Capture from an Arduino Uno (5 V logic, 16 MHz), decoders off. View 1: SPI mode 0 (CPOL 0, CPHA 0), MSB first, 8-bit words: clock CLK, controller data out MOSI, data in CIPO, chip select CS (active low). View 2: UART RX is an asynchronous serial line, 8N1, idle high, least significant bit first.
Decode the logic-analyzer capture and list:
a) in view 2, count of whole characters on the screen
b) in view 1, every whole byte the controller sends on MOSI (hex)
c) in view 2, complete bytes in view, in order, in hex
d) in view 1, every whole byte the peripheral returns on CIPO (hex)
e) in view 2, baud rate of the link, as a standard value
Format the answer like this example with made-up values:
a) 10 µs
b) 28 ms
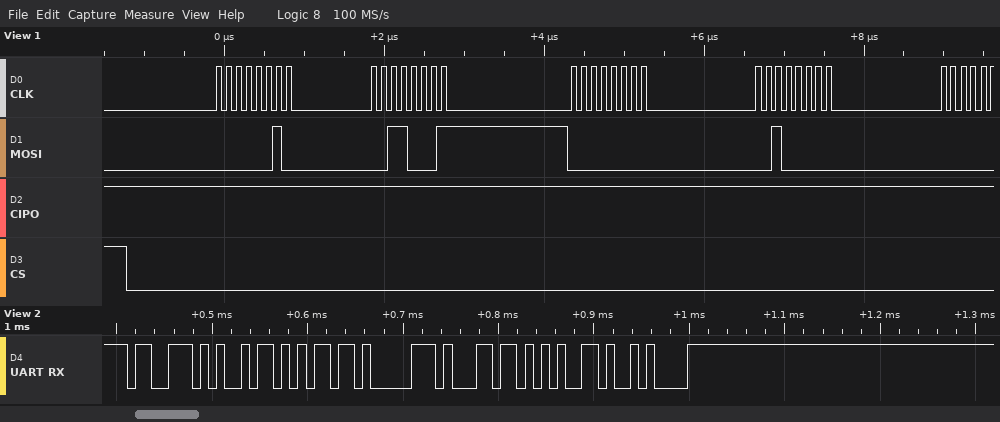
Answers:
a) 7
b) 02 31 00 20
c) 73 69 6D 70 6C 65 0A
d) FF FF FF FF
e) 115200 baud
